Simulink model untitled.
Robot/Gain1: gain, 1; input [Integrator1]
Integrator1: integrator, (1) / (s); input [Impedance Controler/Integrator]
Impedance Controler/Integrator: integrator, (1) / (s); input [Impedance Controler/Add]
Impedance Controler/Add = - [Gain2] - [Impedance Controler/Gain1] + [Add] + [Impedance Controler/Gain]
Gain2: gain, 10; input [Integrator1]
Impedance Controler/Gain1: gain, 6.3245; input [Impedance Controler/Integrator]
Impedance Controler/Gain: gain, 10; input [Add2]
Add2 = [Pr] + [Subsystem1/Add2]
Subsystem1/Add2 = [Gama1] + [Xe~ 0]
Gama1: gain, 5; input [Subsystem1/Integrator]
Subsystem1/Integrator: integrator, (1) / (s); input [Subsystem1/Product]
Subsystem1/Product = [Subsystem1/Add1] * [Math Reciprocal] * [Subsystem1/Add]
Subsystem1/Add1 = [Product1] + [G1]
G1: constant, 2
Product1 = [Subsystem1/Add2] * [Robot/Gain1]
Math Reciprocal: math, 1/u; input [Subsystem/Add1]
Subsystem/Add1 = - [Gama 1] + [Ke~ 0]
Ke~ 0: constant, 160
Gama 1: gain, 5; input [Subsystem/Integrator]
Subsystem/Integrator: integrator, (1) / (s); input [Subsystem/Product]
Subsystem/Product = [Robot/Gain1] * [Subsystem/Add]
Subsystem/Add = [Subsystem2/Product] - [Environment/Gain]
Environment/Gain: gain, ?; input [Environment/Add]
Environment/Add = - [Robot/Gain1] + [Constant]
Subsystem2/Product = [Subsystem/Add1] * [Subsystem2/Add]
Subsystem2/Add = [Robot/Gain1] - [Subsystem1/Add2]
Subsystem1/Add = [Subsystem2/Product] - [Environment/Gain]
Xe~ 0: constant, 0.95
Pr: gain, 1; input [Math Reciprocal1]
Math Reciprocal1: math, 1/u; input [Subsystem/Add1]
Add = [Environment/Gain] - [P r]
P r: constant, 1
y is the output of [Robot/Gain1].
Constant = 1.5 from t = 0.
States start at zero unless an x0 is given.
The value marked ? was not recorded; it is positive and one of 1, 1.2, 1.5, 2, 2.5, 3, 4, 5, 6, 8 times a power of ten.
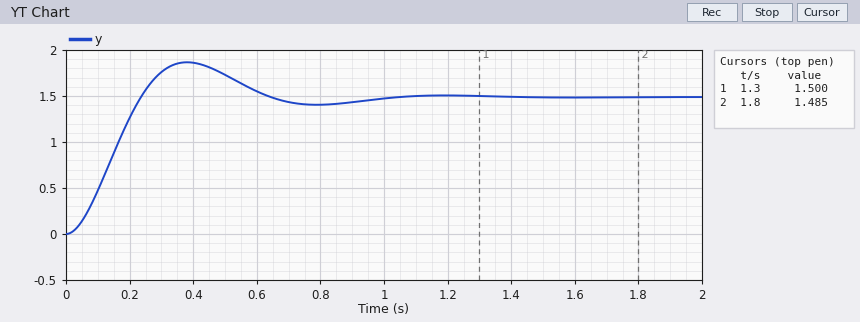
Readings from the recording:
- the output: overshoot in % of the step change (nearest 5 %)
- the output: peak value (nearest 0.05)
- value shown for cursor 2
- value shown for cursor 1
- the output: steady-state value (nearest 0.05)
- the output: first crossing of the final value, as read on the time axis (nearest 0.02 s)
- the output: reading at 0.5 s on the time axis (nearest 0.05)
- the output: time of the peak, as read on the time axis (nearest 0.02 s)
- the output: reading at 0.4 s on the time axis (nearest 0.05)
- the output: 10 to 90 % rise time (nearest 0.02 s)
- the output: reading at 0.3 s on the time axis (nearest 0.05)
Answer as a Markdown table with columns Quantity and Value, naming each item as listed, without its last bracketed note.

| Quantity | Value |
|---|---|
| the output: overshoot in % of the step change | 25 % |
| the output: peak value | 1.85 |
| value shown for cursor 2 | 1.485 |
| value shown for cursor 1 | 1.500 |
| the output: steady-state value | 1.50 |
| the output: first crossing of the final value, as read on the time axis | 0.24 s |
| the output: reading at 0.5 s on the time axis | 1.75 |
| the output: time of the peak, as read on the time axis | 0.38 s |
| the output: reading at 0.4 s on the time axis | 1.85 |
| the output: 10 to 90 % rise time | 0.16 s |
| the output: reading at 0.3 s on the time axis | 1.75 |
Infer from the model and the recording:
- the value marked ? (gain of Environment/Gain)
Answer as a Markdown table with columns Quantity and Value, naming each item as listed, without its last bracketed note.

| Quantity | Value |
|---|---|
| the value marked ? | 80 |
